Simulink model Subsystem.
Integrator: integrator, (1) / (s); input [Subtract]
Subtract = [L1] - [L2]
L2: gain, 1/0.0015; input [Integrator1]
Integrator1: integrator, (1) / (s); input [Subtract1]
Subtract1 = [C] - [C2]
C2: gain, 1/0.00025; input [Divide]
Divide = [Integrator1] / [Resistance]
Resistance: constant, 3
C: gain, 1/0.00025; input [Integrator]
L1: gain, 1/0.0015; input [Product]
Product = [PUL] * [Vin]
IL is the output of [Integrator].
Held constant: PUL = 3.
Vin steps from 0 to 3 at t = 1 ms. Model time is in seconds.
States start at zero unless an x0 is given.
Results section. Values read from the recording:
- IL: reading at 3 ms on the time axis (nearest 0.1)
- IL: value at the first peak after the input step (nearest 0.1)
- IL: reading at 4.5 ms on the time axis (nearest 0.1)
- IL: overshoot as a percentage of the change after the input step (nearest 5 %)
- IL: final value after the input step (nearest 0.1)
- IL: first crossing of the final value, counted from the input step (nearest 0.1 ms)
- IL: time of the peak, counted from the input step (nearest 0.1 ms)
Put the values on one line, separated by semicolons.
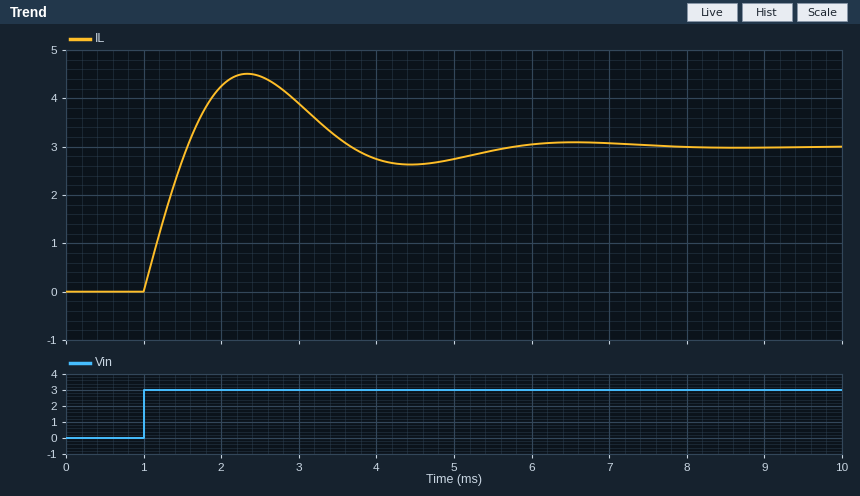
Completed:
3.9; 4.5; 2.6; 50 %; 3.0; 0.6 ms; 1.3 ms
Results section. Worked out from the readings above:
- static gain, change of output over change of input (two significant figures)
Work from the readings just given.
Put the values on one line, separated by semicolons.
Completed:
1.0
